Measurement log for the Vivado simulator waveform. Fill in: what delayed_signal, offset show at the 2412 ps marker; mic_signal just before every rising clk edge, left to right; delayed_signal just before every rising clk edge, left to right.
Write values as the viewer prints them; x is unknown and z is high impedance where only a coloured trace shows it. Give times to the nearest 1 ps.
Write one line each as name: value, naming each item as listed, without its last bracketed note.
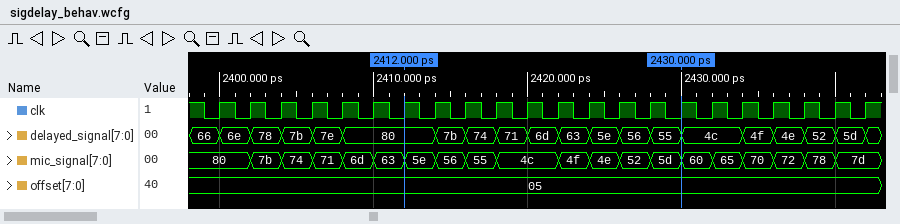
what delayed_signal, offset show at the 2412 ps marker: delayed_signal=80, offset=05
mic_signal just before every rising clk edge, left to right: 80, 80, 7b, 74, 71, 6d, 63, 5e, 56, 55, 4c, 4c, 4f, 4e, 52, 5d, 60, 65, 70, 72, 78, 7d
delayed_signal just before every rising clk edge, left to right: 66, 6e, 78, 7b, 7e, 80, 80, 80, 7b, 74, 71, 6d, 63, 5e, 56, 55, 4c, 4c, 4f, 4e, 52, 5d
